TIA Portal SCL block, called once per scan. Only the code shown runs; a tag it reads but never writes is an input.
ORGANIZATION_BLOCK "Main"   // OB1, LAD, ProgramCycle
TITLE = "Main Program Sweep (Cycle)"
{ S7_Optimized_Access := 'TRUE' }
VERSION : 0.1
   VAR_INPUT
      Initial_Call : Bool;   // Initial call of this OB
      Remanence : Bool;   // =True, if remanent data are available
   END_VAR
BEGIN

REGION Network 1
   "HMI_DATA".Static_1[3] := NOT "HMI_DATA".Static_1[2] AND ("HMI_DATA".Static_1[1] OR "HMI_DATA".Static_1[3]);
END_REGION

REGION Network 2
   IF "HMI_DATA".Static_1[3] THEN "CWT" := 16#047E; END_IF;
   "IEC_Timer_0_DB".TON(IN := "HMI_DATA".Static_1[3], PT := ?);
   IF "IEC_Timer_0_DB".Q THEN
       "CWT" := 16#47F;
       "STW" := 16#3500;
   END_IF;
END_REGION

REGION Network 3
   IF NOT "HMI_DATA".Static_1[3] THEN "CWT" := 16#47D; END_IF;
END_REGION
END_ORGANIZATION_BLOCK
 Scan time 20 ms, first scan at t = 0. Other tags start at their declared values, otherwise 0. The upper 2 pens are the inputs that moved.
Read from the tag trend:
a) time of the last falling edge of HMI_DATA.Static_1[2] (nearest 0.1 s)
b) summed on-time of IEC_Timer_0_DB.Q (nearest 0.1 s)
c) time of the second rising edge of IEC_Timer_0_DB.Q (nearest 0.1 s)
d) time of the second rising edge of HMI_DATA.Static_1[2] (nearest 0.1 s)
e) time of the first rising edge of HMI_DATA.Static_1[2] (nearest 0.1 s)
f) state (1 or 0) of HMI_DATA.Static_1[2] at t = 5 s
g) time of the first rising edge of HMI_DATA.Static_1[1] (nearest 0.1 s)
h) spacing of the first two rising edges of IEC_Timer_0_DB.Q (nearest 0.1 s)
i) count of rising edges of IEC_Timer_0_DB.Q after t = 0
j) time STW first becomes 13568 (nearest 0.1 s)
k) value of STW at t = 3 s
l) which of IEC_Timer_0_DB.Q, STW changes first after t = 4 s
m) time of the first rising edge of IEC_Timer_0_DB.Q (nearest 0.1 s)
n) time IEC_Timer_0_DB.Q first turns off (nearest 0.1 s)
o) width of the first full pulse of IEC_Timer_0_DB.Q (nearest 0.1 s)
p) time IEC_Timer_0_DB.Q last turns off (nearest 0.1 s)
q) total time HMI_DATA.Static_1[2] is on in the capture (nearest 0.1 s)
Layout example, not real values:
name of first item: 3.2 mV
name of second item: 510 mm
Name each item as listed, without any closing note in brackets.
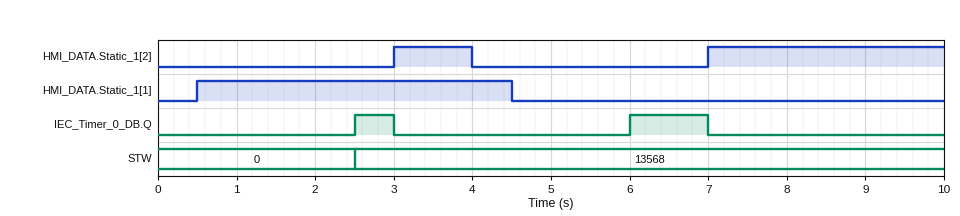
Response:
time of the last falling edge of HMI_DATA.Static_1[2]: 4.0 s
summed on-time of IEC_Timer_0_DB.Q: 1.5 s
time of the second rising edge of IEC_Timer_0_DB.Q: 6.0 s
time of the second rising edge of HMI_DATA.Static_1[2]: 7.0 s
time of the first rising edge of HMI_DATA.Static_1[2]: 3.0 s
state (1 or 0) of HMI_DATA.Static_1[2] at t = 5 s: 0
time of the first rising edge of HMI_DATA.Static_1[1]: 0.5 s
spacing of the first two rising edges of IEC_Timer_0_DB.Q: 3.5 s
count of rising edges of IEC_Timer_0_DB.Q after t = 0: 2
time STW first becomes 13568: 2.5 s
value of STW at t = 3 s: 13568
which of IEC_Timer_0_DB.Q, STW changes first after t = 4 s: IEC_Timer_0_DB.Q
time of the first rising edge of IEC_Timer_0_DB.Q: 2.5 s
time IEC_Timer_0_DB.Q first turns off: 3.0 s
width of the first full pulse of IEC_Timer_0_DB.Q: 0.5 s
time IEC_Timer_0_DB.Q last turns off: 7.0 s
total time HMI_DATA.Static_1[2] is on in the capture: 4.0 s
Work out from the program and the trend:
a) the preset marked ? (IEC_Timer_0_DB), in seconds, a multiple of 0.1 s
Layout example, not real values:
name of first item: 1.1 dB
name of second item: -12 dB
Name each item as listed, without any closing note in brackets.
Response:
the preset marked ? (IEC_Timer_0_DB), in seconds, a multiple of 0.1 s: 2.0 s
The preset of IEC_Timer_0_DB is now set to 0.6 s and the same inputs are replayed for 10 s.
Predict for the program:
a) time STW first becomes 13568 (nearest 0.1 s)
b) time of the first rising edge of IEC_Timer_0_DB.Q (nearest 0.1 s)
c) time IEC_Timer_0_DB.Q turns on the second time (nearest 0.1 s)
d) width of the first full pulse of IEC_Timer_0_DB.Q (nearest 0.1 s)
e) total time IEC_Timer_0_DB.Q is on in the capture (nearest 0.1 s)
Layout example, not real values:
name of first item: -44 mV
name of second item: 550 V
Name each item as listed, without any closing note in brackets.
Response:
time STW first becomes 13568: 1.1 s
time of the first rising edge of IEC_Timer_0_DB.Q: 1.1 s
time IEC_Timer_0_DB.Q turns on the second time: 4.6 s
width of the first full pulse of IEC_Timer_0_DB.Q: 1.9 s
total time IEC_Timer_0_DB.Q is on in the capture: 4.3 s
